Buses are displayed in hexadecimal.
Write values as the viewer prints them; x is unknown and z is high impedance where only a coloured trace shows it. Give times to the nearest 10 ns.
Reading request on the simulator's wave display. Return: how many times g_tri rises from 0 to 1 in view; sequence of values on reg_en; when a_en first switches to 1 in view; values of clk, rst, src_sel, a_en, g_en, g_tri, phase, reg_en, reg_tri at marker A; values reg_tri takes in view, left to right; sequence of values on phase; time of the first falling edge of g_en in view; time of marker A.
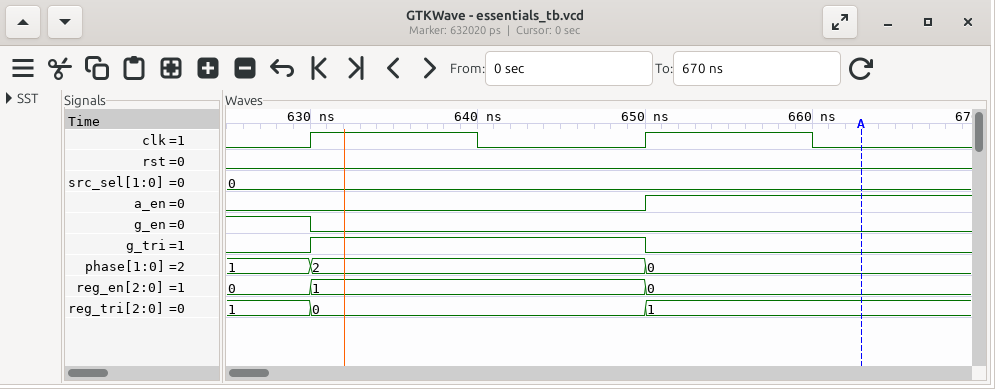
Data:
1
0, 1, 0
650 ns
clk=0, rst=0, src_sel=0, a_en=1, g_en=0, g_tri=0, phase=0, reg_en=0, reg_tri=1
1, 0, 1
1, 2, 0
630 ns
660 ns
